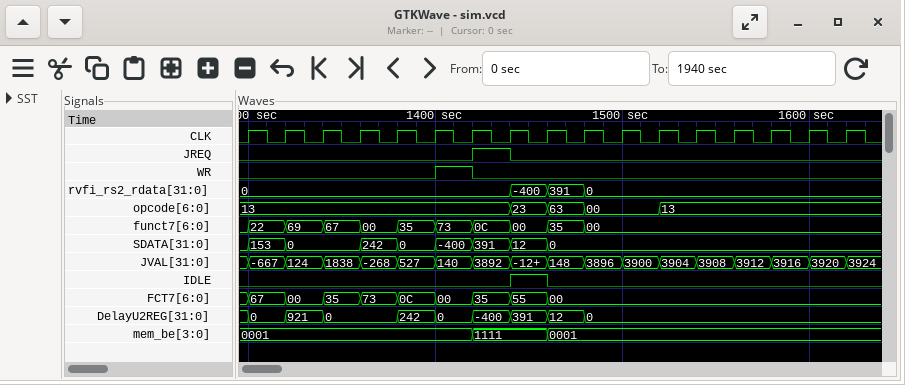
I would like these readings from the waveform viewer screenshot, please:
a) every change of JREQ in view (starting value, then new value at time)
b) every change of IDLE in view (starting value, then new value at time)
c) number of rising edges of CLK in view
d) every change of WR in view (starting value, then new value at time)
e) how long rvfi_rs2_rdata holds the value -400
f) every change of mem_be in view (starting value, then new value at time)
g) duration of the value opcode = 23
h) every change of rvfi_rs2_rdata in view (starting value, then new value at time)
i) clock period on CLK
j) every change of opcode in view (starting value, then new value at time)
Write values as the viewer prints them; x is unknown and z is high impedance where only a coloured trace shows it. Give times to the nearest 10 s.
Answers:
0, 1 at 1420 s, 0 at 1440 s
0, 1 at 1440 s, 0 at 1460 s
17
0, 1 at 1400 s, 0 at 1420 s
20 s
0001, 1111 at 1420 s, 0001 at 1460 s
20 s
0, -400 at 1440 s, 391 at 1460 s, 0 at 1480 s
20 s
13, 23 at 1440 s, 63 at 1460 s, 00 at 1480 s, 13 at 1520 s
